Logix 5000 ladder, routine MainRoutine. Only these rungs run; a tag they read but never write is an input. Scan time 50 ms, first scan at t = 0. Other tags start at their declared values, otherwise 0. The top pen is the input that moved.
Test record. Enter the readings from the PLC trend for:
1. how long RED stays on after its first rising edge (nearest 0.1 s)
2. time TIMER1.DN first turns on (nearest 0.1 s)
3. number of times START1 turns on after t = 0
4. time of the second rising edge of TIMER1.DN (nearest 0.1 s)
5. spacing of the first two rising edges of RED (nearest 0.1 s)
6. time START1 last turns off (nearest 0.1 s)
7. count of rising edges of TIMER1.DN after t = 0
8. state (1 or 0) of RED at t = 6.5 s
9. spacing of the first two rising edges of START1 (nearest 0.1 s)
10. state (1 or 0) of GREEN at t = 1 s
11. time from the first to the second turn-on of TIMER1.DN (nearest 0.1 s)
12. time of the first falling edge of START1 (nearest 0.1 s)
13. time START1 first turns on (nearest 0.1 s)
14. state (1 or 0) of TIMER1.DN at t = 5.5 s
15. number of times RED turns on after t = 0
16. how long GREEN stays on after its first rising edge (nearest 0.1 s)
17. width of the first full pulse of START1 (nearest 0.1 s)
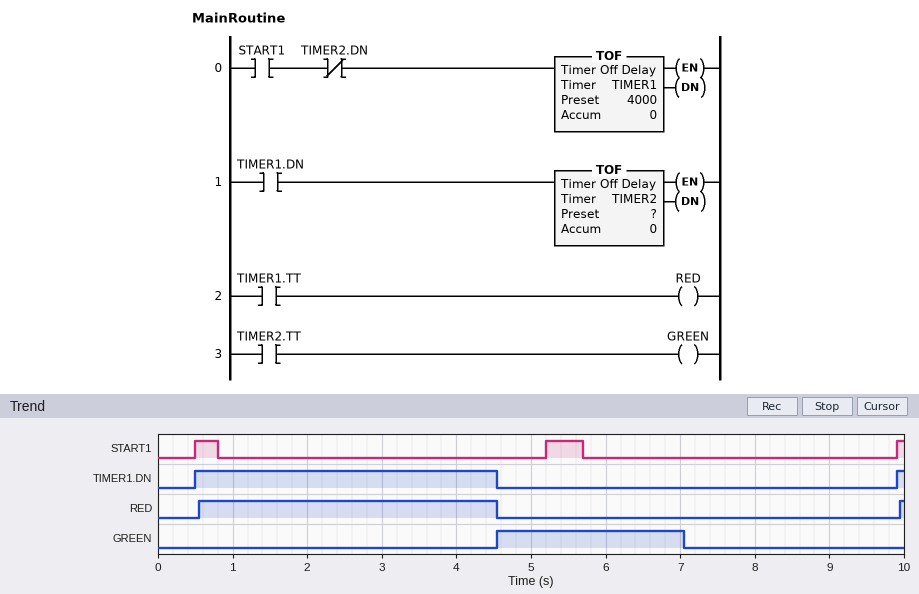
4.0 s
0.5 s
3
9.9 s
9.4 s
5.7 s
2
0
4.7 s
0
9.4 s
0.8 s
0.5 s
0
2
2.5 s
0.3 s
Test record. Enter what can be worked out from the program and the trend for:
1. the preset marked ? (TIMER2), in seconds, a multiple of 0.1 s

2.5 s
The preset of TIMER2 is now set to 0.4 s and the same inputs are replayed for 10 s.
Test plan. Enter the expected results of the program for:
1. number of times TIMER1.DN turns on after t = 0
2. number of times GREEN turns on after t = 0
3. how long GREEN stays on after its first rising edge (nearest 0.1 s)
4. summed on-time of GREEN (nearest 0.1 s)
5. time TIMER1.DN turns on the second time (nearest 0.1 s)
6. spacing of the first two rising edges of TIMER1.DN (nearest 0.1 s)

3
2
0.4 s
0.8 s
5.2 s
4.7 s
